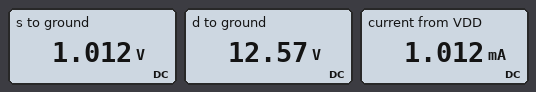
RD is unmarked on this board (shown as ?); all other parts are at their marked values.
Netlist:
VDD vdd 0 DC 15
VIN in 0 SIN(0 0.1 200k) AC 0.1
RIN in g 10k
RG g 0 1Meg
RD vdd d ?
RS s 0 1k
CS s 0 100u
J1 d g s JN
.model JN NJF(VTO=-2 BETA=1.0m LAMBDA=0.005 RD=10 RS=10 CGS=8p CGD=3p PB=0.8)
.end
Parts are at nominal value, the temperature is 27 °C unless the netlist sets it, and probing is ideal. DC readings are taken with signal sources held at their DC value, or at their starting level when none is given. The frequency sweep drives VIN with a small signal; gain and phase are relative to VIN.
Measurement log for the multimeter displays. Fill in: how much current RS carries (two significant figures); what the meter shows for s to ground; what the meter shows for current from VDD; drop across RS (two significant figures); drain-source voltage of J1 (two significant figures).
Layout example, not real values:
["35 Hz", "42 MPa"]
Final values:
["1.0 mA", "1.012 V", "1.012 mA", "1.0 V", "12 V"]
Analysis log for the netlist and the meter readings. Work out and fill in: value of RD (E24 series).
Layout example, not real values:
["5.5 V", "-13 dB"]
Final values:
["2.4 kΩ"]
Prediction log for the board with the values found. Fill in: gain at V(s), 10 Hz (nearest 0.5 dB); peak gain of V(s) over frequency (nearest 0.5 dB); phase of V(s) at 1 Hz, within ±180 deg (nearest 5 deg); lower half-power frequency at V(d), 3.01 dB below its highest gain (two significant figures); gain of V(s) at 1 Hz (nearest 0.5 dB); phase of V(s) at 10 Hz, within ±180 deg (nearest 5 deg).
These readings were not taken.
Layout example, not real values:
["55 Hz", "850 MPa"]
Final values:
["-11.0 dB", "-3.5 dB", "-10 deg", "4.2 Hz", "-4.0 dB", "-65 deg"]
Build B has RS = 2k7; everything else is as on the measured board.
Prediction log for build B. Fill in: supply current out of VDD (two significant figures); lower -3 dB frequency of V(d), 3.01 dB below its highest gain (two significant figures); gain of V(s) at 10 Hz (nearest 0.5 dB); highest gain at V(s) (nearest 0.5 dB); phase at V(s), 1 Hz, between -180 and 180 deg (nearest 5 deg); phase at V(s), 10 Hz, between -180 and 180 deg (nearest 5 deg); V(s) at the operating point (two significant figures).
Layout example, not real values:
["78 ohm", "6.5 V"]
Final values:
["490 µA", "2.7 Hz", "-13.5 dB", "-2.0 dB", "-20 deg", "-75 deg", "1.3 V"]
